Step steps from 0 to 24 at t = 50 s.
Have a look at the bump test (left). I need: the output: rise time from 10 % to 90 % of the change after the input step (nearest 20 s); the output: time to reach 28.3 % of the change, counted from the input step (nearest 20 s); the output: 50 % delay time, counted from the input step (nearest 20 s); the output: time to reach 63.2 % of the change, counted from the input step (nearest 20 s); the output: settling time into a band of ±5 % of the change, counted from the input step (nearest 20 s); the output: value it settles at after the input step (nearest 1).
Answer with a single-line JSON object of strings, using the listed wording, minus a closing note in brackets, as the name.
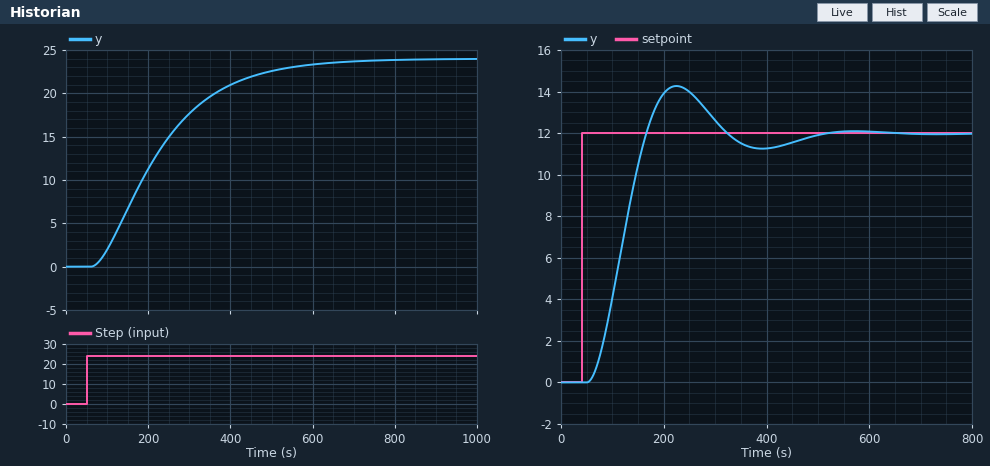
{"the output: rise time from 10 % to 90 % of the change after the input step": "320 s", "the output: time to reach 28.3 % of the change, counted from the input step": "100 s", "the output: 50 % delay time, counted from the input step": "160 s", "the output: time to reach 63.2 % of the change, counted from the input step": "200 s", "the output: settling time into a band of ±5 % of the change, counted from the input step": "480 s", "the output: value it settles at after the input step": "24"}
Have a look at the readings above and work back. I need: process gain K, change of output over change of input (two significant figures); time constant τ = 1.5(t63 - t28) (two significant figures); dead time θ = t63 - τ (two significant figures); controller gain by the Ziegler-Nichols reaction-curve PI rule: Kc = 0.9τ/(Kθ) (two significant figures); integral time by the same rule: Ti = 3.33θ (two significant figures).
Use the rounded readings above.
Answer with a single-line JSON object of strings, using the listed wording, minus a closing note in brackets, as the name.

{"process gain K, change of output over change of input": "1.0", "time constant τ = 1.5(t63 - t28)": "150 s", "dead time θ = t63 - τ": "50 s", "controller gain by the Ziegler-Nichols reaction-curve PI rule: Kc = 0.9τ/(Kθ)": "2.7", "integral time by the same rule: Ti = 3.33θ": "170 s"}
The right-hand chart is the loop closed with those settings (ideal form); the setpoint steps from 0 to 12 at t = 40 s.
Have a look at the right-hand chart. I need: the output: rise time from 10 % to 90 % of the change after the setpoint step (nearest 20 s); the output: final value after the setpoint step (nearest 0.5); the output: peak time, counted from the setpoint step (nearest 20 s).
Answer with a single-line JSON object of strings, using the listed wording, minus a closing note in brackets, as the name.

{"the output: rise time from 10 % to 90 % of the change after the setpoint step": "80 s", "the output: final value after the setpoint step": "12.0", "the output: peak time, counted from the setpoint step": "180 s"}
